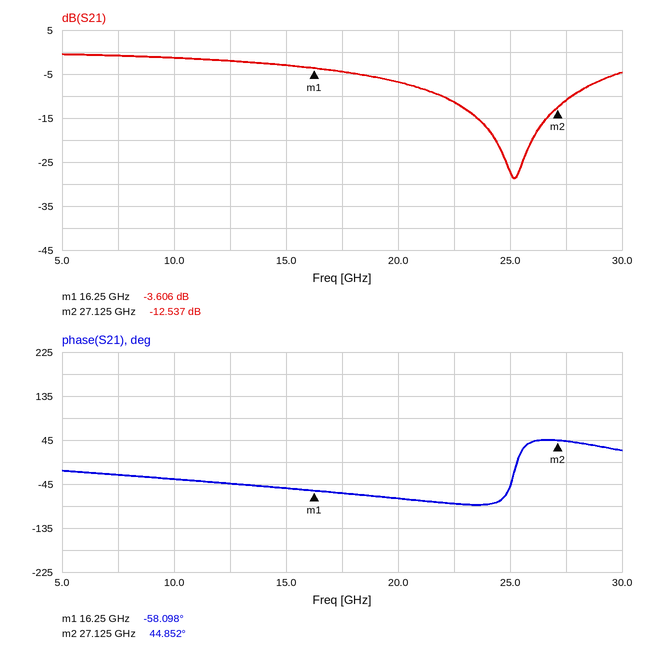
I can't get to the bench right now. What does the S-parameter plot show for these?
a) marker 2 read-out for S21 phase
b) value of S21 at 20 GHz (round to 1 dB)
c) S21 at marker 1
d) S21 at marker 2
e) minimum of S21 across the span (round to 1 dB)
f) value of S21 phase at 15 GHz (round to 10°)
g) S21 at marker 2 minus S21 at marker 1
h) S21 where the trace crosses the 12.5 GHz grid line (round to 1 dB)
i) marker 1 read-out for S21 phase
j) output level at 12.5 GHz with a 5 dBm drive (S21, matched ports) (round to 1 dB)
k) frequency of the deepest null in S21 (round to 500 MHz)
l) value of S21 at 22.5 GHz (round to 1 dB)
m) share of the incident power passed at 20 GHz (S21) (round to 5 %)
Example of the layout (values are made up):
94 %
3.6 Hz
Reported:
44.852°
-7 dB
-3.606 dB
-12.537 dB
-29 dB
-50°
-8.931 dB
-2 dB
-58.098°
3 dBm
25.0 GHz
-11 dB
20 %
